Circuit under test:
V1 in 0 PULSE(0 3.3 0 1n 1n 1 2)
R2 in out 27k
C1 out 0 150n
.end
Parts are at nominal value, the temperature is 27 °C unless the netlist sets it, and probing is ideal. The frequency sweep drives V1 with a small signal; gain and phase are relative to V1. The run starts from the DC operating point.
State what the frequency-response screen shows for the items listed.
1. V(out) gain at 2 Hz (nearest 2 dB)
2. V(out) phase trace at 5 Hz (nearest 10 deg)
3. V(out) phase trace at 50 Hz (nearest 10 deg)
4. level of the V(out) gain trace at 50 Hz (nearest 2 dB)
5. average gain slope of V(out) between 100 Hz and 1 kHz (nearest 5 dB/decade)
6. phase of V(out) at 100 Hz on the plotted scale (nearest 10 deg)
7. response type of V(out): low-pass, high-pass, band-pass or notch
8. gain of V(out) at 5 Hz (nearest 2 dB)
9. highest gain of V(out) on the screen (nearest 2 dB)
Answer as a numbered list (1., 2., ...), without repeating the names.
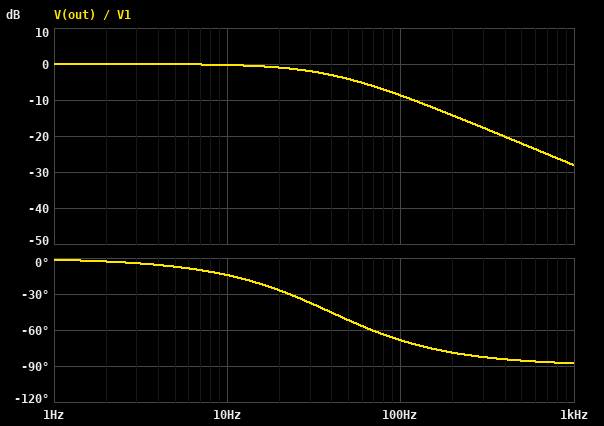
1. 0 dB
2. -10 deg
3. -50 deg
4. -4 dB
5. -20 dB/decade
6. -70 deg
7. low-pass
8. 0 dB
9. 0 dB
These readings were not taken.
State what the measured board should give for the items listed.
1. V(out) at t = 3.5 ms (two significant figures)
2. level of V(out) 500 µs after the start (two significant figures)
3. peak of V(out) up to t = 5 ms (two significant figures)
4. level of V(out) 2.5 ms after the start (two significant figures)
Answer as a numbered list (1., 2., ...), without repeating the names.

1. 1.9 V
2. 380 mV
3. 2.3 V
4. 1.5 V
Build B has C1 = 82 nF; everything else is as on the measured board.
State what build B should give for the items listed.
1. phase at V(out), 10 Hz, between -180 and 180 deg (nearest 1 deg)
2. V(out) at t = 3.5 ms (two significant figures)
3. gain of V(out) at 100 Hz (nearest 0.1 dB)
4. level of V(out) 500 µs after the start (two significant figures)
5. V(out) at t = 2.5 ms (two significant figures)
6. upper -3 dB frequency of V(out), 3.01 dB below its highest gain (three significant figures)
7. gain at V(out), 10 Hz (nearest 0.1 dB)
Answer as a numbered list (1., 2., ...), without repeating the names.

1. -8 deg
2. 2.6 V
3. -4.7 dB
4. 670 mV
5. 2.2 V
6. 71.9 Hz
7. -0.1 dB
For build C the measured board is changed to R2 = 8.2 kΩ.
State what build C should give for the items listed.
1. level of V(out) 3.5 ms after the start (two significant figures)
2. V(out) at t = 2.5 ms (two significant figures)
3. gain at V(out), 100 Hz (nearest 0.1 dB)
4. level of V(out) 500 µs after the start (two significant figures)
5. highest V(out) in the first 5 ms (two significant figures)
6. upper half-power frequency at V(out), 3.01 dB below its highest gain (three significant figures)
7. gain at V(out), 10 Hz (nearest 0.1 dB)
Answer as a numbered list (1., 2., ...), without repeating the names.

1. 3.1 V
2. 2.9 V
3. -2.0 dB
4. 1.1 V
5. 3.2 V
6. 129 Hz
7. 0 dB
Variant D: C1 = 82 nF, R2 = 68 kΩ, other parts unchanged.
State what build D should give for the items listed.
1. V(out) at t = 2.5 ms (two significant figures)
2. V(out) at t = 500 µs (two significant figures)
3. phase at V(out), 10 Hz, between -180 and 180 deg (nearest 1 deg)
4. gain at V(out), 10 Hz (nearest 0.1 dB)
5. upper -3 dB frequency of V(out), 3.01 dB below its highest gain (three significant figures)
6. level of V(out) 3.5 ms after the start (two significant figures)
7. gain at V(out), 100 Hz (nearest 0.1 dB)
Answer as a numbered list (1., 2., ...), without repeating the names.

1. 1.2 V
2. 280 mV
3. -19 deg
4. -0.5 dB
5. 28.5 Hz
6. 1.5 V
7. -11.2 dB
